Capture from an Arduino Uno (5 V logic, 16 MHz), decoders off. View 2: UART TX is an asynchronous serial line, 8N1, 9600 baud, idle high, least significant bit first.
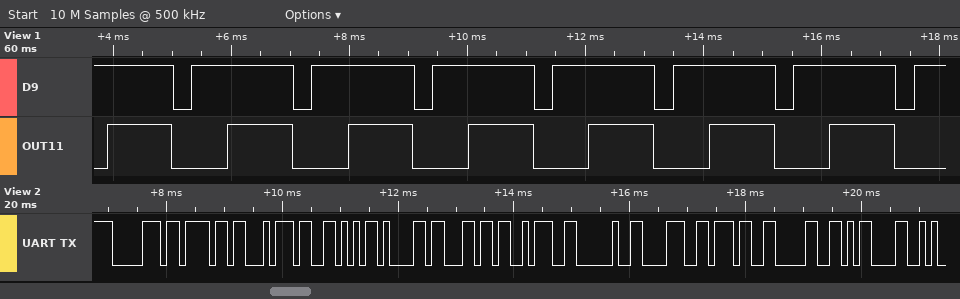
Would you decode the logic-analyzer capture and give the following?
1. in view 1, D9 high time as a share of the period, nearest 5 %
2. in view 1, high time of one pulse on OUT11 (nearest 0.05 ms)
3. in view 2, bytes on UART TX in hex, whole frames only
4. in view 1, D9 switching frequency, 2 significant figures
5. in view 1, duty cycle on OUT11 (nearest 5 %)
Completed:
85 %
1.10 ms
70 6F 74 56 61 6C 3A 20 38 37 30 0D
490 Hz
55 %
